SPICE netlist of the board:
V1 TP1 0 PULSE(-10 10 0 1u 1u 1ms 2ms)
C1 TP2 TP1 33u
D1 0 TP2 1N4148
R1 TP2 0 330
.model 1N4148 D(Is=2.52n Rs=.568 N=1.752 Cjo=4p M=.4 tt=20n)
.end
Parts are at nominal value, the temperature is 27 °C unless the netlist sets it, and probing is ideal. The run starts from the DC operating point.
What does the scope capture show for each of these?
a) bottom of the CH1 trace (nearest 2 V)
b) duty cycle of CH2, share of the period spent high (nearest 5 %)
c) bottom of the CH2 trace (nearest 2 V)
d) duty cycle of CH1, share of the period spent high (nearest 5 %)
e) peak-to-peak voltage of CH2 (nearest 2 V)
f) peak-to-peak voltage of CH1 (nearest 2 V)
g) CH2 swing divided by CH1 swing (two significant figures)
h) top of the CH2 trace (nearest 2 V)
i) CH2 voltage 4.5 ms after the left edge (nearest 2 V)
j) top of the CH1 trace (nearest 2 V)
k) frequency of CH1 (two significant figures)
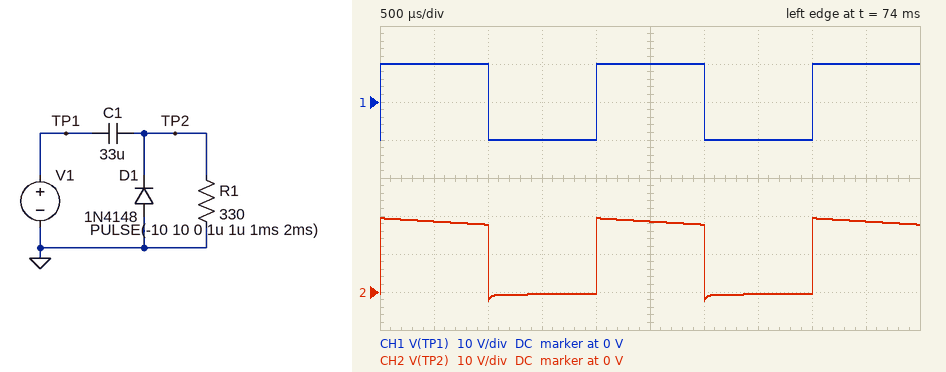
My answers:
-10 V
50 %
-2 V
50 %
22 V
20 V
1.1
20 V
18 V
10 V
500 Hz
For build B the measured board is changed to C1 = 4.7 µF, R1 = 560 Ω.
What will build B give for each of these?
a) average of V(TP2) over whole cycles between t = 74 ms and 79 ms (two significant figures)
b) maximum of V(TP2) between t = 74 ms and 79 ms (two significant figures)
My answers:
7.9 V
20 V
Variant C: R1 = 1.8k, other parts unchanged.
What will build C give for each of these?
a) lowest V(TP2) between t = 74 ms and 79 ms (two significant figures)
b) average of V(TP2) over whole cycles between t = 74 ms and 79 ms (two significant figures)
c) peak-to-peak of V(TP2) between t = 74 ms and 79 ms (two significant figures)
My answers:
-930 mV
9.3 V
20 V
